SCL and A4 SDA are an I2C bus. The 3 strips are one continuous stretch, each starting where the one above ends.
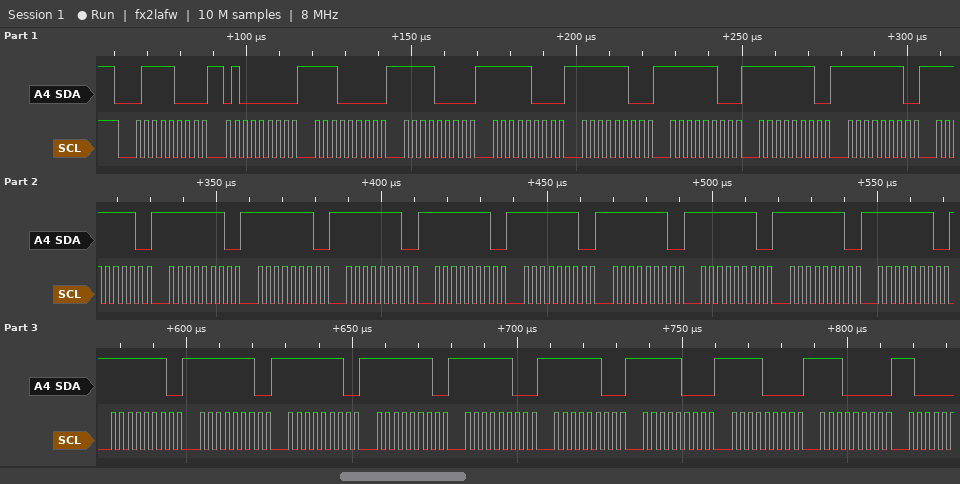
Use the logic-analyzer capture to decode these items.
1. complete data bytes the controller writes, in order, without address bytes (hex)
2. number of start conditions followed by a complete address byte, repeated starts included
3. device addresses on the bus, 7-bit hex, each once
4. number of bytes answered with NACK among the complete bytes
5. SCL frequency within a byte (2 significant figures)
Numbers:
40 E0 F0 F8 FC FC FE FE FE FE FE FE FE FE FE FE FE FE FE FE FE FE FC FC F8 F0 E0
1
0x3C
0
400 kHz
